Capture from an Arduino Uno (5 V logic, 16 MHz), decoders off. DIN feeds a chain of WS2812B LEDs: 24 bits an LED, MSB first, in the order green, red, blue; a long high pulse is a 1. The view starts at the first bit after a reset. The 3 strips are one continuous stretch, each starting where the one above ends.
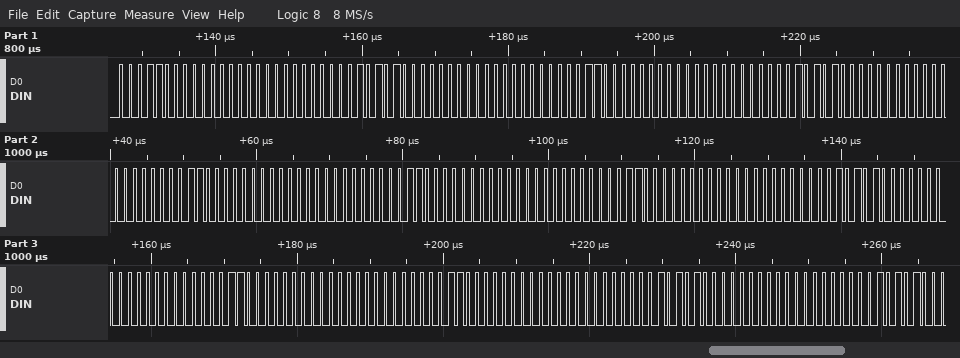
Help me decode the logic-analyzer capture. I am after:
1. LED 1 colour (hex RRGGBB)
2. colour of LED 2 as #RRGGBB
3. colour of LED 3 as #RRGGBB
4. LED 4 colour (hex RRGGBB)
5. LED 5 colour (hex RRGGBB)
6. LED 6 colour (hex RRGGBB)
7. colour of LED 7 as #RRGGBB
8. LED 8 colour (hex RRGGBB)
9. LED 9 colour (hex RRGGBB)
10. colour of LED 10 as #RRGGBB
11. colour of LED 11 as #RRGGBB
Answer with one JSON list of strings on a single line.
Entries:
["#001800", "#002A00", "#001800", "#002A00", "#001800", "#001800", "#001800", "#002A00", "#001800", "#001800", "#002A00"]
